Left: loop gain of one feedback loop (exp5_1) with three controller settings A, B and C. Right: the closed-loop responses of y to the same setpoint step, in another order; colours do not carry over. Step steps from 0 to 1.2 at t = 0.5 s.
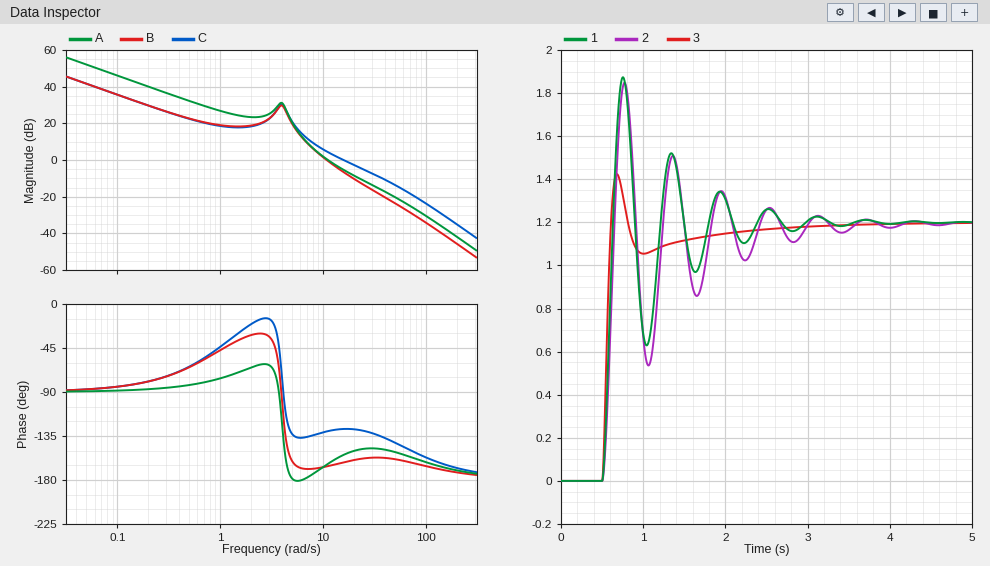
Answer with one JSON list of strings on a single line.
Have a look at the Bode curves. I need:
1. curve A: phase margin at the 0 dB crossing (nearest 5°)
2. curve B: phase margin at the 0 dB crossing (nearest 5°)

["15°", "15°"]
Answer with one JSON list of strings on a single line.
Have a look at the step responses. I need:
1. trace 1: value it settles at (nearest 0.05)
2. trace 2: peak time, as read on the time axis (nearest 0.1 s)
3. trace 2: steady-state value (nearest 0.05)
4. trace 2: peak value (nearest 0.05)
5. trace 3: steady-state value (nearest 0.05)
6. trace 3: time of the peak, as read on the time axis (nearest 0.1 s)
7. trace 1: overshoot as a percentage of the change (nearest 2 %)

["1.20", "0.8 s", "1.20", "1.85", "1.20", "0.7 s", "56 %"]
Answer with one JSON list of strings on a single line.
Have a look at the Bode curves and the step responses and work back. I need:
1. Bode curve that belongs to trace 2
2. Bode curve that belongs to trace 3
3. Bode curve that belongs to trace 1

["B", "C", "A"]
